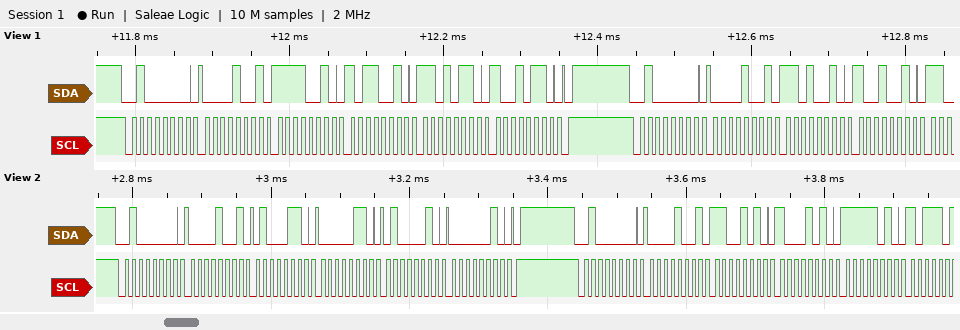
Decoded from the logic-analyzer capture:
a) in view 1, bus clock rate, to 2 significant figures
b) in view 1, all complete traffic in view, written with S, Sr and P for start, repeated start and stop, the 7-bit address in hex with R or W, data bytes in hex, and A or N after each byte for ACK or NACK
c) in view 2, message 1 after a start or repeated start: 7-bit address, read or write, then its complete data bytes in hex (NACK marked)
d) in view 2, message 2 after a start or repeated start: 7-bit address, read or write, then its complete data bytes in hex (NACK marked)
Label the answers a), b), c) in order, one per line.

a) 100 kHz
b) S 20W A 09 A F2 A B2 A D6 A 96 A P S 20W A 09 A D2 A 92 A
c) 0x20 write: 09 46 06 42 02
d) 0x20 write: 09 CA 8A FA
